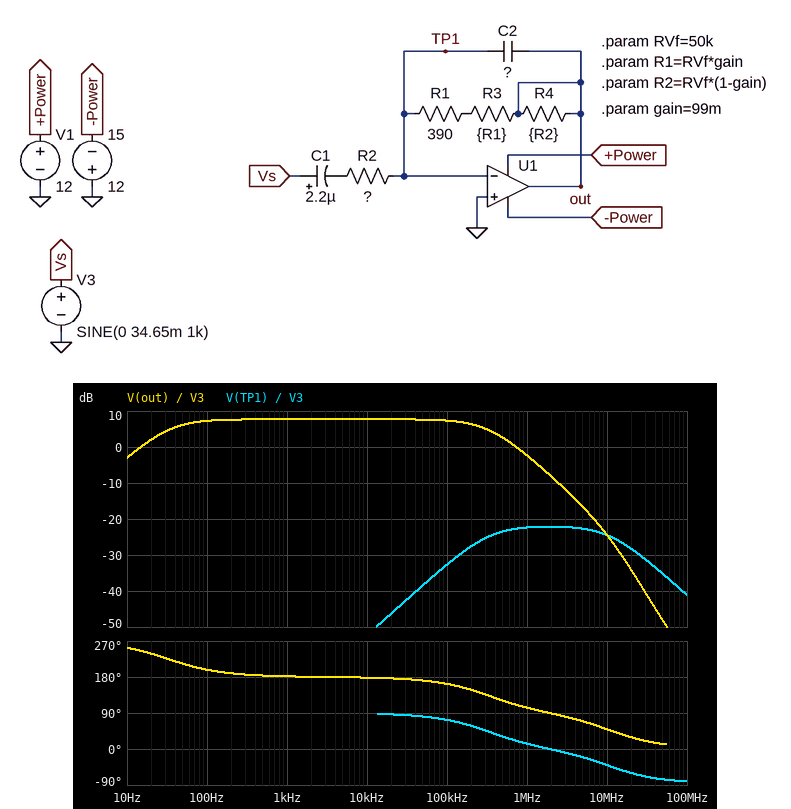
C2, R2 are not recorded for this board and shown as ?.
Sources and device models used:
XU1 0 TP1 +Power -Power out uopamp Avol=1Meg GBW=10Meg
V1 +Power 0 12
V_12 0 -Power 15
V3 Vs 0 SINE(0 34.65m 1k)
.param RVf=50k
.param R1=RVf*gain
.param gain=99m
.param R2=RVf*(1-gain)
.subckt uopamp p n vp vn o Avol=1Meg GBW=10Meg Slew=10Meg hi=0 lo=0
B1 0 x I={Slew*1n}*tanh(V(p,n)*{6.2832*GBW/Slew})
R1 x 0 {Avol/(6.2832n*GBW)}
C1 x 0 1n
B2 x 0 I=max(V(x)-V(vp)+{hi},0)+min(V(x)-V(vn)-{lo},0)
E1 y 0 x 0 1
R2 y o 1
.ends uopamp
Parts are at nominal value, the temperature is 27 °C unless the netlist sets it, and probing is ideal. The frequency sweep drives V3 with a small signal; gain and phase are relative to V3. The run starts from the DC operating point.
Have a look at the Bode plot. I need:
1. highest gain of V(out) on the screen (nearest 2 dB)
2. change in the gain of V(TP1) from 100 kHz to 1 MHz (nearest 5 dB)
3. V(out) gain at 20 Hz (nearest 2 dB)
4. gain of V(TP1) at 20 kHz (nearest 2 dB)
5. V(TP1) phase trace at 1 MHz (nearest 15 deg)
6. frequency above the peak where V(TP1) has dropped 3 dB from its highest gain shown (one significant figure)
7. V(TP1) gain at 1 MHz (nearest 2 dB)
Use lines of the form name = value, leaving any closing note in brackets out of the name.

highest gain of V(out) on the screen = 8 dB
change in the gain of V(TP1) from 100 kHz to 1 MHz = 10 dB
V(out) gain at 20 Hz = 2 dB
gain of V(TP1) at 20 kHz = -46 dB
V(TP1) phase trace at 1 MHz = 15 deg
frequency above the peak where V(TP1) has dropped 3 dB from its highest gain shown = 10 MHz
V(TP1) gain at 1 MHz = -22 dB
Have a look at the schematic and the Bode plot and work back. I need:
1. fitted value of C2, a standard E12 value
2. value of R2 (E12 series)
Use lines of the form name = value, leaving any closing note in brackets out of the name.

fitted value of C2, a standard E12 value = 82 pF
value of R2 = 2.2 kΩ
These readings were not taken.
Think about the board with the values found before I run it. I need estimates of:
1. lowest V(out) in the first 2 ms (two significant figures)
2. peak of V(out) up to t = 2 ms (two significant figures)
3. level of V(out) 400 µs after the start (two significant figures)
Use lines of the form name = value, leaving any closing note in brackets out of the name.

lowest V(out) in the first 2 ms = -82 mV
peak of V(out) up to t = 2 ms = 86 mV
level of V(out) 400 µs after the start = -45 mV
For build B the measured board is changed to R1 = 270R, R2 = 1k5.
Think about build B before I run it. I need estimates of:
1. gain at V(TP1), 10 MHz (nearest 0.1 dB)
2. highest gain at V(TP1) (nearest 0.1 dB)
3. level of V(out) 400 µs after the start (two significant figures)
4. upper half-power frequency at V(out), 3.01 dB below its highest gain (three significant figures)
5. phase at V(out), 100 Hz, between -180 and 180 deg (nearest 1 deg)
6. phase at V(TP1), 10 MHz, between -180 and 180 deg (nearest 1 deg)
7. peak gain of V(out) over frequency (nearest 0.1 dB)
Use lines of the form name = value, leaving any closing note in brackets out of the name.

gain at V(TP1), 10 MHz = -21.4 dB
highest gain at V(TP1) = -19.1 dB
level of V(out) 400 µs after the start = -61 mV
upper half-power frequency at V(out), 3.01 dB below its highest gain = 328 kHz
phase at V(out), 100 Hz, between -180 and 180 deg = -154 deg
phase at V(TP1), 10 MHz, between -180 and 180 deg = -39 deg
peak gain of V(out) over frequency = 10.8 dB
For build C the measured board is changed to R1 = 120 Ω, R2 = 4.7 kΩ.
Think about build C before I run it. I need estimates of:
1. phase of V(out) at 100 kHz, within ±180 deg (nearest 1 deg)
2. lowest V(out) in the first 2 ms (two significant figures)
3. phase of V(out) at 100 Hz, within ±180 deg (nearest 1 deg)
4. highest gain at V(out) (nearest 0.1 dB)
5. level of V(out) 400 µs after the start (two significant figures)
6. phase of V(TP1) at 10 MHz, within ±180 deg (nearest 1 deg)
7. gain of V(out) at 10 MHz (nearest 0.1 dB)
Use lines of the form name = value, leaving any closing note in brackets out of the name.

phase of V(out) at 100 kHz, within ±180 deg = 164 deg
lowest V(out) in the first 2 ms = -37 mV
phase of V(out) at 100 Hz, within ±180 deg = -171 deg
highest gain at V(out) = 0.7 dB
level of V(out) 400 µs after the start = -21 mV
phase of V(TP1) at 10 MHz, within ±180 deg = -41 deg
gain of V(out) at 10 MHz = -30.8 dB
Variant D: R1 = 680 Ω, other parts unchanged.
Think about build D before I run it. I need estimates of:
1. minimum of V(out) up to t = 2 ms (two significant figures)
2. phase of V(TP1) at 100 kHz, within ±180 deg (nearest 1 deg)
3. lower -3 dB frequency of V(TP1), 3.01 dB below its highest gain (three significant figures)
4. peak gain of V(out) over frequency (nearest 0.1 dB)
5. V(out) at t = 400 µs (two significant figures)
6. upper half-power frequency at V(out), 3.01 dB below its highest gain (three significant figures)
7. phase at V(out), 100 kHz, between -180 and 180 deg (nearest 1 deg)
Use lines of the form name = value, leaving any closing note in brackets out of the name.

minimum of V(out) up to t = 2 ms = -86 mV
phase of V(TP1) at 100 kHz, within ±180 deg = 72 deg
lower -3 dB frequency of V(TP1), 3.01 dB below its highest gain = 299 kHz
peak gain of V(out) over frequency = 8.2 dB
V(out) at t = 400 µs = -47 mV
upper half-power frequency at V(out), 3.01 dB below its highest gain = 316 kHz
phase at V(out), 100 kHz, between -180 and 180 deg = 162 deg
